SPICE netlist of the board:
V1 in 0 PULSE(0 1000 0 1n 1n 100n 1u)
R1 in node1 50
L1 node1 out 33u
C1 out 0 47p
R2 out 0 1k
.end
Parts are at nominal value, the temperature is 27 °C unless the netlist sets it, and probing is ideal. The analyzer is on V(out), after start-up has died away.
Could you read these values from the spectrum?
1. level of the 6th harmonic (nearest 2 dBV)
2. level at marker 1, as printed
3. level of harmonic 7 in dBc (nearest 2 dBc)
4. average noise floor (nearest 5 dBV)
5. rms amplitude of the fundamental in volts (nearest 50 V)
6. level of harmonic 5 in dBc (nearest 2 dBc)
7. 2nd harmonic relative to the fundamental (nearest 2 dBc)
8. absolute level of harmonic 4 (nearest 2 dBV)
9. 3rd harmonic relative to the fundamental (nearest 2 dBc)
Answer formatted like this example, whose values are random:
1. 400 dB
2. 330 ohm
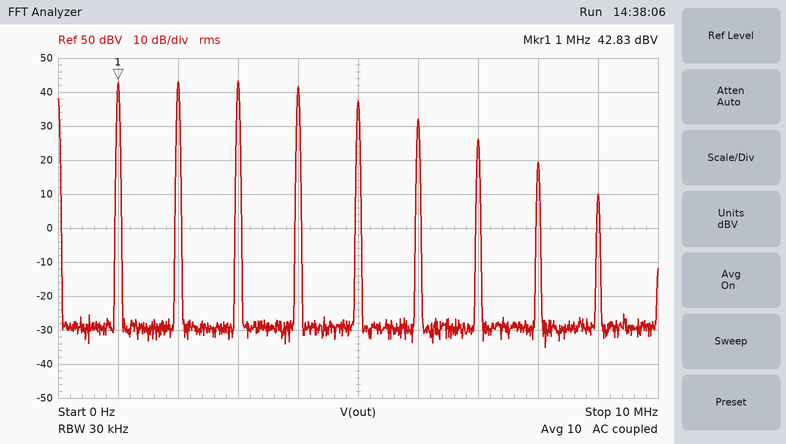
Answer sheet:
1. 32 dBV
2. 42.83 dBV
3. -16 dBc
4. -30 dBV
5. 150 V
6. -6 dBc
7. 0 dBc
8. 42 dBV
9. 0 dBc
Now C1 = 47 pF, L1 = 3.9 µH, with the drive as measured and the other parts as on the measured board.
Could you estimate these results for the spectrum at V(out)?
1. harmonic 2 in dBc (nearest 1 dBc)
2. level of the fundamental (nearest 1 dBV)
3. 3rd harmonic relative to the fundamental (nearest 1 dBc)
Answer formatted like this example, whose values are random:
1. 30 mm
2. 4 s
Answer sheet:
1. 0 dBc
2. 43 dBV
3. -1 dBc
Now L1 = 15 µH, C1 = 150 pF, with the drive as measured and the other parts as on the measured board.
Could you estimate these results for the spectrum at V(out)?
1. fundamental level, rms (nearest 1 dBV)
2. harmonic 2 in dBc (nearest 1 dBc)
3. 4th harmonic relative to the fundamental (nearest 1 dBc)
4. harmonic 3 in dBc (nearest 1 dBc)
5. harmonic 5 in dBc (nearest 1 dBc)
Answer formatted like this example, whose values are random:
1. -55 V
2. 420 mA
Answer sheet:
1. 43 dBV
2. 2 dBc
3. 1 dBc
4. 5 dBc
5. -7 dBc
